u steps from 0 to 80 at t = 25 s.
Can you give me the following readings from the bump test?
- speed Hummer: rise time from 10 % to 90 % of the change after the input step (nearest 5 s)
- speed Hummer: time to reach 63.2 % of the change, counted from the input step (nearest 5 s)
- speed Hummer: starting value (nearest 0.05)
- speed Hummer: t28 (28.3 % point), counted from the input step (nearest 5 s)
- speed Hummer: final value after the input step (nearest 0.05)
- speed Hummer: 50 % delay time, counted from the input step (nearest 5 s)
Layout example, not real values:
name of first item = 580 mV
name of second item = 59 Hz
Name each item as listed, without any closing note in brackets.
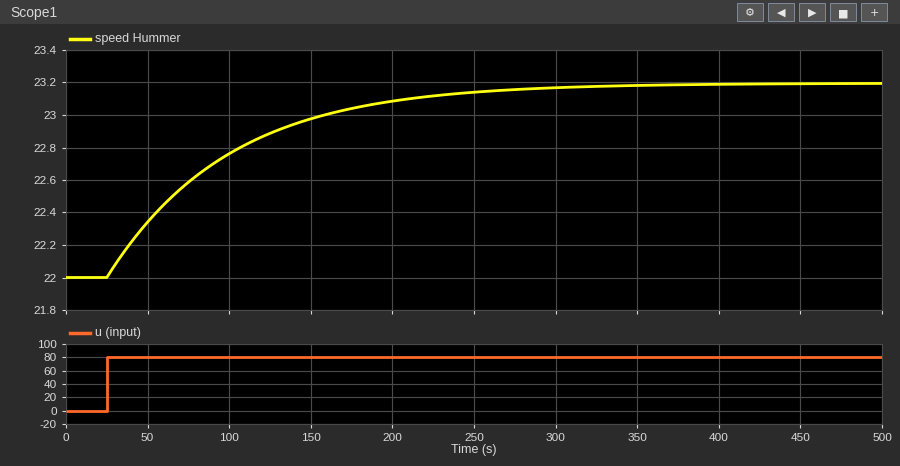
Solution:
speed Hummer: rise time from 10 % to 90 % of the change after the input step = 160 s
speed Hummer: time to reach 63.2 % of the change, counted from the input step = 75 s
speed Hummer: starting value = 22.00
speed Hummer: t28 (28.3 % point), counted from the input step = 25 s
speed Hummer: final value after the input step = 23.20
speed Hummer: 50 % delay time, counted from the input step = 50 s
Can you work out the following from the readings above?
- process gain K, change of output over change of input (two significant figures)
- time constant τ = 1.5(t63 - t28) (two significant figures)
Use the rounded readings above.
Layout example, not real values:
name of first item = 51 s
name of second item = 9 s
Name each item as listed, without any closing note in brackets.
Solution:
process gain K, change of output over change of input = 0.015
time constant τ = 1.5(t63 - t28) = 75 s
